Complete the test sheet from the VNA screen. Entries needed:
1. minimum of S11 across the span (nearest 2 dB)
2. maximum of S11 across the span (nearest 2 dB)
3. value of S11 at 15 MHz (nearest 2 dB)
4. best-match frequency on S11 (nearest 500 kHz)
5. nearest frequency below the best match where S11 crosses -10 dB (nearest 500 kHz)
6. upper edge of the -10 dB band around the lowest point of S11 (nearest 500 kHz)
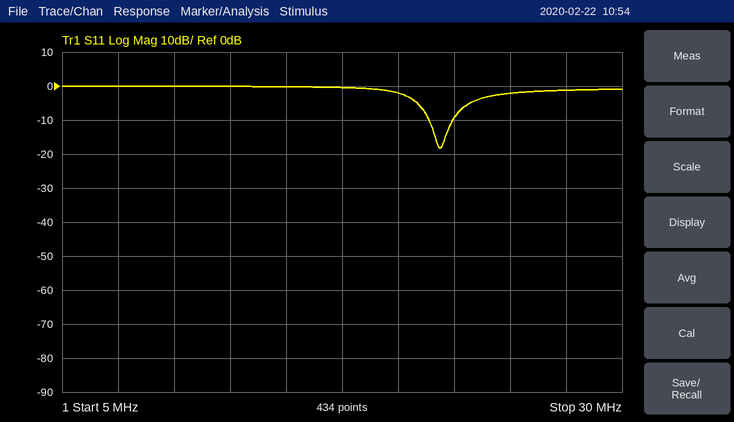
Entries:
-18 dB
0 dB
0 dB
22.0 MHz
21.5 MHz
22.5 MHz
